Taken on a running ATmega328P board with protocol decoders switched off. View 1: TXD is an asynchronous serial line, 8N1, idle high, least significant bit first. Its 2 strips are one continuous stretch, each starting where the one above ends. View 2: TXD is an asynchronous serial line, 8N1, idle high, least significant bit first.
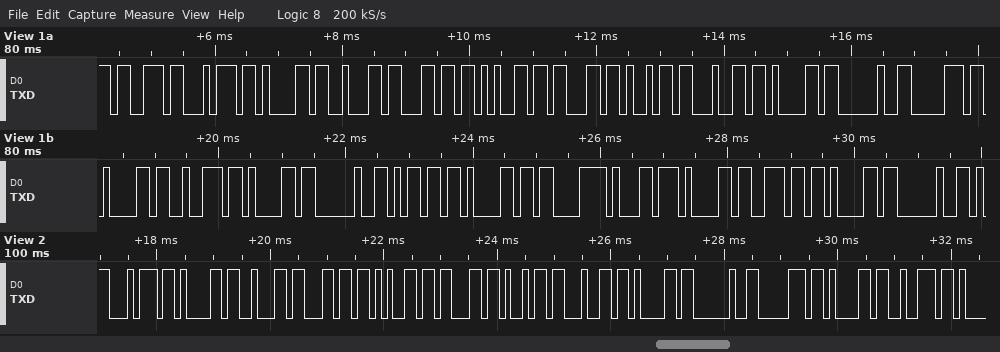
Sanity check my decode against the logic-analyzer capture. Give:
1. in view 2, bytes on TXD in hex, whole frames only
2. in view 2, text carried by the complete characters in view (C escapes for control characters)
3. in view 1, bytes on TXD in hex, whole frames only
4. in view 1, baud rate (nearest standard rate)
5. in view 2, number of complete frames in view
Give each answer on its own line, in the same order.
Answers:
74 61 62 6C 65 63 69 64 61 20 70 61 72
"tablecida par"
0x73 0x74 0x61 0x62 0x6C 0x65 0x63 0x69 0x64 0x61 0x20 0x70 0x61 0x72 0x61 0x20 0x6D 0x61 0xC3 0xB1 0x61 0x6E 0x61 0x20
9600 baud
13
